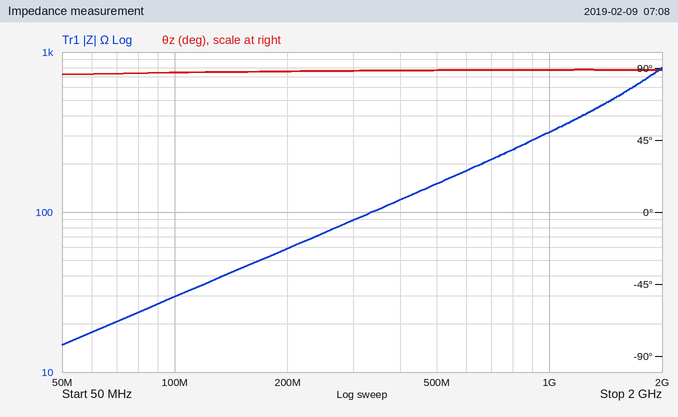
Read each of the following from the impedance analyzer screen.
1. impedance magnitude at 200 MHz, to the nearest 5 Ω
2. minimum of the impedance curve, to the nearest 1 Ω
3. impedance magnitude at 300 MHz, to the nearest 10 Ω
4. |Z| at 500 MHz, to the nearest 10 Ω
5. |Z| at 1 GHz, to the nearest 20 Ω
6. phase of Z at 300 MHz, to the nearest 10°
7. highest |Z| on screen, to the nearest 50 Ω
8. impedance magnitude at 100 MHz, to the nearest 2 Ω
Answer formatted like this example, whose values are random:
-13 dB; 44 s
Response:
60 Ω; 15 Ω; 90 Ω; 150 Ω; 320 Ω; 90°; 800 Ω; 30 Ω
